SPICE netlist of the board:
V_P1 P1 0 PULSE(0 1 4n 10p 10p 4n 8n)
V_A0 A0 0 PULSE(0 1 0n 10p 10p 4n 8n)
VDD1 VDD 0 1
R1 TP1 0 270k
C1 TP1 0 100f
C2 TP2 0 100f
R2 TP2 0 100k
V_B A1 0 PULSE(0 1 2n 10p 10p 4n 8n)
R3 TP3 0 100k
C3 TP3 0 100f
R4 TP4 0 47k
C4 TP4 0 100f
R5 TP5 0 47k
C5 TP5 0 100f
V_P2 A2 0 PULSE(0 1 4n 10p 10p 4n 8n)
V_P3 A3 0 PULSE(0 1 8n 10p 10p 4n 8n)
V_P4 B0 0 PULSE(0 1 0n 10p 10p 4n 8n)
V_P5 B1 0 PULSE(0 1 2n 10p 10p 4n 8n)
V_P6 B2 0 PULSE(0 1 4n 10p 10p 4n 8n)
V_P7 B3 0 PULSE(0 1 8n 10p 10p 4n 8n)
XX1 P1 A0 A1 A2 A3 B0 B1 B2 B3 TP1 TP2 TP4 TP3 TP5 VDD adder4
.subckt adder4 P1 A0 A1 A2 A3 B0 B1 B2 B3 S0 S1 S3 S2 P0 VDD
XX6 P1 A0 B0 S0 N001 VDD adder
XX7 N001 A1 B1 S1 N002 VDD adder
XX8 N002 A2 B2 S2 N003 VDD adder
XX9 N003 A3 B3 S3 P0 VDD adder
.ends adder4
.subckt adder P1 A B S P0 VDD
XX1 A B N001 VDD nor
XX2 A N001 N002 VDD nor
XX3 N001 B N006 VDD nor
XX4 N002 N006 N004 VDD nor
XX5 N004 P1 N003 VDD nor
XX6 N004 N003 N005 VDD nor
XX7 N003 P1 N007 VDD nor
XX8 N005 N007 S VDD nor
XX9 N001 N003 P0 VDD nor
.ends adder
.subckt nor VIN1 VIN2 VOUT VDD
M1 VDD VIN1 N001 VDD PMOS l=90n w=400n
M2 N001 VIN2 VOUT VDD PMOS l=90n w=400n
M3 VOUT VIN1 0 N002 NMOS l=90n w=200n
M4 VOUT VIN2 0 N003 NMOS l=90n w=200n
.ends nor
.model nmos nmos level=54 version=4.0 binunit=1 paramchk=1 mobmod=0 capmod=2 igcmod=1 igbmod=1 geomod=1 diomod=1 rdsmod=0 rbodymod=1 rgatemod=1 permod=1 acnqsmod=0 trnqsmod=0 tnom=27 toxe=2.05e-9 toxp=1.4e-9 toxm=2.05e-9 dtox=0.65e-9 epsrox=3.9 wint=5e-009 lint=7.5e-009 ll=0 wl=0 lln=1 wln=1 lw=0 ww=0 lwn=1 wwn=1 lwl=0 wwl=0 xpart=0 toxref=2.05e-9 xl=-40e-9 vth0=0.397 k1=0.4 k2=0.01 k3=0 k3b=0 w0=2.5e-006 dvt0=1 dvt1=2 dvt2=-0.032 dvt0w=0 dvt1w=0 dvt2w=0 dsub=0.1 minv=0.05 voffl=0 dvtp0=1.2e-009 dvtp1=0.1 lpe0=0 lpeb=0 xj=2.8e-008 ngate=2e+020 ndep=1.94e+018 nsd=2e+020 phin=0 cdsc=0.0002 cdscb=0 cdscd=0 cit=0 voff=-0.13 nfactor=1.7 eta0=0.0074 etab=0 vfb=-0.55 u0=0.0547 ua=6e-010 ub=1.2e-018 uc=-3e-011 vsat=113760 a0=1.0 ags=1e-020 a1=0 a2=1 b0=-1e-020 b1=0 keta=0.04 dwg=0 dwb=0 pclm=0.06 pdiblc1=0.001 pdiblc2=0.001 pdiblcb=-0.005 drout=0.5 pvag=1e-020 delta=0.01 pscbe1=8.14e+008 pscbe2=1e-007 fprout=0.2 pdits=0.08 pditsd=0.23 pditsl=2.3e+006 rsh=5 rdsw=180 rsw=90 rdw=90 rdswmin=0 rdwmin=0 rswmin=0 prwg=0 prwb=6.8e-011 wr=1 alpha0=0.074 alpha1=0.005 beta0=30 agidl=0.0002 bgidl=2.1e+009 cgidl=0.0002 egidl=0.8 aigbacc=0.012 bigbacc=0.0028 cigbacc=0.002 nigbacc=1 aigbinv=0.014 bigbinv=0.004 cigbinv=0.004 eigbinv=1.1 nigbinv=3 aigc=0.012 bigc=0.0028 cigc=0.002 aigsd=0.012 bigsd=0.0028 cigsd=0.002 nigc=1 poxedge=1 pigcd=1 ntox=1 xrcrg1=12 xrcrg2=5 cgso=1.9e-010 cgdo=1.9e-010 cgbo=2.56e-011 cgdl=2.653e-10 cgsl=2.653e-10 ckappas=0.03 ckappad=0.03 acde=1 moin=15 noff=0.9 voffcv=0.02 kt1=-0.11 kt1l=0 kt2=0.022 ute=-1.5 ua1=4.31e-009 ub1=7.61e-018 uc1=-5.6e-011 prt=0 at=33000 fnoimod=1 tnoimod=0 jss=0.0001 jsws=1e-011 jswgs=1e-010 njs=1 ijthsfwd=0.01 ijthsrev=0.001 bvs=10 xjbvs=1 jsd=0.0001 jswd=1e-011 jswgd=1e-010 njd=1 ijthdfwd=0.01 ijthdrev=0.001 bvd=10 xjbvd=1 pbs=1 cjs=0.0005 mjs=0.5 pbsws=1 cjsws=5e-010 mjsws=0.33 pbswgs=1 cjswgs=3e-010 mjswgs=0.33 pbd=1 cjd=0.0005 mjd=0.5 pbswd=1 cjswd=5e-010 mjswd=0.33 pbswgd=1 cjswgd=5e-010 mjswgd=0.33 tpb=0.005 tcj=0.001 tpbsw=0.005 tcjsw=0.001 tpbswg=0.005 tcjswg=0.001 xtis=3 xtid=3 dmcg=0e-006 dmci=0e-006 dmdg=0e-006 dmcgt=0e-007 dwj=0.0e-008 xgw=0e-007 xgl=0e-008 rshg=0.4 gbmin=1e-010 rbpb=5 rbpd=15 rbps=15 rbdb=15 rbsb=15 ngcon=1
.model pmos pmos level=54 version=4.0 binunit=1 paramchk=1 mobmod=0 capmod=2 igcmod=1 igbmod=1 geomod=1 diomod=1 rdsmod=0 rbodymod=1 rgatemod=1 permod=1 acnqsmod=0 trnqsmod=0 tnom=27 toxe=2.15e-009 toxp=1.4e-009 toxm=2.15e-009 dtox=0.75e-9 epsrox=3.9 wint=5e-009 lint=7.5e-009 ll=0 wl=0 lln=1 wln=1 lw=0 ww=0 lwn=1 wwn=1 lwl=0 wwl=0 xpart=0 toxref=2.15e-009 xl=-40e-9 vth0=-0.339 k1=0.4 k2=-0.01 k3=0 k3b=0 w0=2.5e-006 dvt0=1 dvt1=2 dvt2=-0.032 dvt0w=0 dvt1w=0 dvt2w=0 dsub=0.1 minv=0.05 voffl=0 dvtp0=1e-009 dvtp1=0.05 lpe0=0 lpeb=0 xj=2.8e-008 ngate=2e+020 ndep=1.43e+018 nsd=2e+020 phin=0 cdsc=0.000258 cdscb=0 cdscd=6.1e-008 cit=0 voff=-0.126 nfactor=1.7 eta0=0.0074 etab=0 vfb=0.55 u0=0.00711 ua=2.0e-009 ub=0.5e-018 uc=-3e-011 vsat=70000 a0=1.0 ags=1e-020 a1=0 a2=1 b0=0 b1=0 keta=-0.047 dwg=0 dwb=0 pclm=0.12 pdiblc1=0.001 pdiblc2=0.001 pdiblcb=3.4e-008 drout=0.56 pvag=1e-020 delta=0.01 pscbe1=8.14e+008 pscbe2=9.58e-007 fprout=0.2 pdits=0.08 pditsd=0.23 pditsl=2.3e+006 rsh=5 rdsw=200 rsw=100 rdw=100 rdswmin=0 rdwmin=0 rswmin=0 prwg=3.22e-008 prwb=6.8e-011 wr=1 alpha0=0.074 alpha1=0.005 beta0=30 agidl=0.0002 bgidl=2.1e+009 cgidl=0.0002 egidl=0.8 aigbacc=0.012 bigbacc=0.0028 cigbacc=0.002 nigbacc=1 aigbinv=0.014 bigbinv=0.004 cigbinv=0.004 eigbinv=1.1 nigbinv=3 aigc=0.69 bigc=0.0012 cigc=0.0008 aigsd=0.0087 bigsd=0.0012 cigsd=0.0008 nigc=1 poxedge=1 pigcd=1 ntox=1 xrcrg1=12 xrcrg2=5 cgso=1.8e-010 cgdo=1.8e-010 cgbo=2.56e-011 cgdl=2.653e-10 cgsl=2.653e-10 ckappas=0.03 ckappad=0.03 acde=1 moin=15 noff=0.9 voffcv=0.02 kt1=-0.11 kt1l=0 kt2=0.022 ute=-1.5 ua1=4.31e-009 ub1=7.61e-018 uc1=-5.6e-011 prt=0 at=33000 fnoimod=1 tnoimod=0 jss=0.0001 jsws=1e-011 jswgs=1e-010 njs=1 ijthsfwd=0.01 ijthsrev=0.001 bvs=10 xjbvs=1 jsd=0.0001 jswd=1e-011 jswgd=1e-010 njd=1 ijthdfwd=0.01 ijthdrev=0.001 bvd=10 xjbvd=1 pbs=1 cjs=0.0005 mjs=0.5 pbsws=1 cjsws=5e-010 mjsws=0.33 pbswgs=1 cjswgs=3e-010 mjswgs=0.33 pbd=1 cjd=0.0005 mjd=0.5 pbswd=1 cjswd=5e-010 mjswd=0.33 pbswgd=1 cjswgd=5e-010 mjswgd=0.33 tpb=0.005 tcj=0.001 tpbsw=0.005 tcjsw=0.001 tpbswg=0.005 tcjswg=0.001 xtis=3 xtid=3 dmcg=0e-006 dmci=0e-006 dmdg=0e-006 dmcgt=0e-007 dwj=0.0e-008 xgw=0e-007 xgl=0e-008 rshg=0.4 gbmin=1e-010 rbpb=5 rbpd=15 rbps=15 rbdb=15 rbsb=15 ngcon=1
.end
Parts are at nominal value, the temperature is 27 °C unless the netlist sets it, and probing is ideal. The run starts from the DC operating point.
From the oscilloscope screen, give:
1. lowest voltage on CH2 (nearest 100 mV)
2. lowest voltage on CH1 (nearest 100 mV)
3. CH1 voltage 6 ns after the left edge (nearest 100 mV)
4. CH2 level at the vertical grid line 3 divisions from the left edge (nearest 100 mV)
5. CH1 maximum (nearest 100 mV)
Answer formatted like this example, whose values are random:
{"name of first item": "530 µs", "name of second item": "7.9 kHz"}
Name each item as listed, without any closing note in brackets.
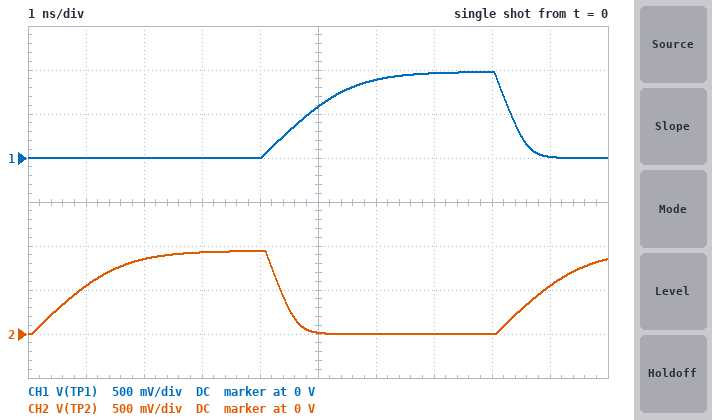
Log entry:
{"lowest voltage on CH2": "0 V", "lowest voltage on CH1": "0 V", "CH1 voltage 6 ns after the left edge": "900 mV", "CH2 level at the vertical grid line 3 divisions from the left edge": "900 mV", "CH1 maximum": "1.0 V"}
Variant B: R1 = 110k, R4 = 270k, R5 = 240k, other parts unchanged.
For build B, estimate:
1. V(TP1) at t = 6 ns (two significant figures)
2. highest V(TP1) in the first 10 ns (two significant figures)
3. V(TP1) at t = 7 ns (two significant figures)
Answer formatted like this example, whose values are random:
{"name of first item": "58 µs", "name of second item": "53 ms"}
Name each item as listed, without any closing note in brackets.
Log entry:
{"V(TP1) at t = 6 ns": "860 mV", "highest V(TP1) in the first 10 ns": "950 mV", "V(TP1) at t = 7 ns": "930 mV"}
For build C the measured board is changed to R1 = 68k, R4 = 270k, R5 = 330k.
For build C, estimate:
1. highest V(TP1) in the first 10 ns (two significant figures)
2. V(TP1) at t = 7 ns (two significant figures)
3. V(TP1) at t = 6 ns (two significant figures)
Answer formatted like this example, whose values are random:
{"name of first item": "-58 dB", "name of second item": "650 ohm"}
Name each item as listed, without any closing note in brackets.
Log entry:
{"highest V(TP1) in the first 10 ns": "920 mV", "V(TP1) at t = 7 ns": "900 mV", "V(TP1) at t = 6 ns": "830 mV"}
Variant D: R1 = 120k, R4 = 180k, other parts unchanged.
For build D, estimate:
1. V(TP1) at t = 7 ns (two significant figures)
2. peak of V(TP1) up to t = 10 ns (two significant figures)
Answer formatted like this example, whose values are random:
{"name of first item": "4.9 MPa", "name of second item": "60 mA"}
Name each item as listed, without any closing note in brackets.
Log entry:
{"V(TP1) at t = 7 ns": "940 mV", "peak of V(TP1) up to t = 10 ns": "950 mV"}
